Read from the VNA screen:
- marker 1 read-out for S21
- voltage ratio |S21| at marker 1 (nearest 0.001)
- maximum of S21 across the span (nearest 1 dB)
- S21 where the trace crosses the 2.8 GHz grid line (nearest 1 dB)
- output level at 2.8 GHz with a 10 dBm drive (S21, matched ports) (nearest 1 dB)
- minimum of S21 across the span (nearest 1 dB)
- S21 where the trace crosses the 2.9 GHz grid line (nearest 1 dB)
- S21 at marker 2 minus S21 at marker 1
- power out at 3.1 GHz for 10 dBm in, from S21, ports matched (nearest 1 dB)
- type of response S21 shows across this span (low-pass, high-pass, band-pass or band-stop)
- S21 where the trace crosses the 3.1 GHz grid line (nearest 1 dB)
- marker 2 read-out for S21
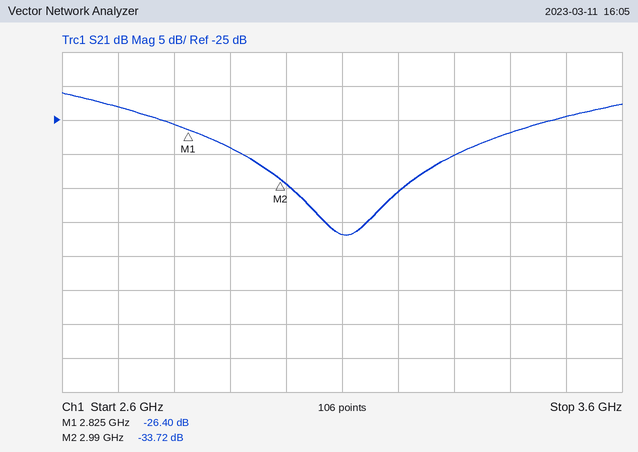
-26.40 dB
0.048
-21 dB
-26 dB
-16 dBm
-42 dB
-29 dB
-7.32 dB
-32 dBm
band-stop
-42 dB
-33.72 dB
